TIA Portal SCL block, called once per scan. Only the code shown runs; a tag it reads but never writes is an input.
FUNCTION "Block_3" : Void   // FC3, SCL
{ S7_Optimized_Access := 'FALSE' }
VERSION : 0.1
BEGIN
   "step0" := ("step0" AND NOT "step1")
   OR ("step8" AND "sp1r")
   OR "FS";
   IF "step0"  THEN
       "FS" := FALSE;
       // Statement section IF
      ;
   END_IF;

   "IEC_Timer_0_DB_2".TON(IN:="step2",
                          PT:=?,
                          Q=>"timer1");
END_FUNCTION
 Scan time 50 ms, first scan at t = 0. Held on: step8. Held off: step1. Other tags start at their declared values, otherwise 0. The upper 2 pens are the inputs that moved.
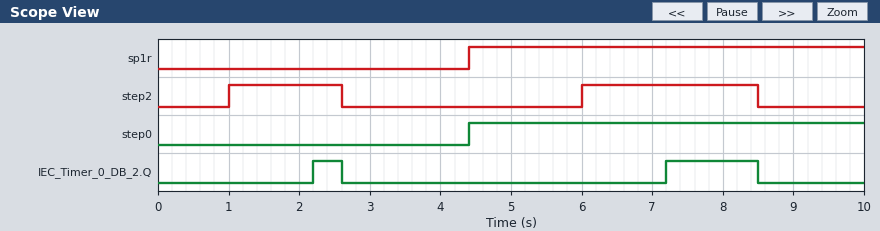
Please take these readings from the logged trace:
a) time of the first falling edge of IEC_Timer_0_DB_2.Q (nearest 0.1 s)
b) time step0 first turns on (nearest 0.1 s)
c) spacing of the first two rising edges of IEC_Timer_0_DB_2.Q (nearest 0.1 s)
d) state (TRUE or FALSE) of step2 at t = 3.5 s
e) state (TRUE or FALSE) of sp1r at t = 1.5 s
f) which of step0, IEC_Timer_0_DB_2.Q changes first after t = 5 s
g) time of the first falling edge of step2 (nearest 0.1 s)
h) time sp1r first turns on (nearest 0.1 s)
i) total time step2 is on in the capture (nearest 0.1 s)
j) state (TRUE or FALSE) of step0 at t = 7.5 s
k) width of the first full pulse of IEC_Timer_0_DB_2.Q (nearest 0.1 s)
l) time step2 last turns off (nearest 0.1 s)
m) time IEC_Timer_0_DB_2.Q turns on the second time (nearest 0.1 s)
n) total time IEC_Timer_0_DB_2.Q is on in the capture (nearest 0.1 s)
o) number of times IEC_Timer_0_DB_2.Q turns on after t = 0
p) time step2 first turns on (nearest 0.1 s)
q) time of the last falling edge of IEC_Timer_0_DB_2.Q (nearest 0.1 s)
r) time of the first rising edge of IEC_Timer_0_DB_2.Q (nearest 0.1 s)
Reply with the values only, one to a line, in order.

2.6 s
4.4 s
5.0 s
FALSE
FALSE
IEC_Timer_0_DB_2.Q
2.6 s
4.4 s
4.1 s
TRUE
0.4 s
8.5 s
7.2 s
1.7 s
2
1.0 s
8.5 s
2.2 s
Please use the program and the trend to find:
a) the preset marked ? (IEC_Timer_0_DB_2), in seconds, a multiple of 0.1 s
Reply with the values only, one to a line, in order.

1.2 s
